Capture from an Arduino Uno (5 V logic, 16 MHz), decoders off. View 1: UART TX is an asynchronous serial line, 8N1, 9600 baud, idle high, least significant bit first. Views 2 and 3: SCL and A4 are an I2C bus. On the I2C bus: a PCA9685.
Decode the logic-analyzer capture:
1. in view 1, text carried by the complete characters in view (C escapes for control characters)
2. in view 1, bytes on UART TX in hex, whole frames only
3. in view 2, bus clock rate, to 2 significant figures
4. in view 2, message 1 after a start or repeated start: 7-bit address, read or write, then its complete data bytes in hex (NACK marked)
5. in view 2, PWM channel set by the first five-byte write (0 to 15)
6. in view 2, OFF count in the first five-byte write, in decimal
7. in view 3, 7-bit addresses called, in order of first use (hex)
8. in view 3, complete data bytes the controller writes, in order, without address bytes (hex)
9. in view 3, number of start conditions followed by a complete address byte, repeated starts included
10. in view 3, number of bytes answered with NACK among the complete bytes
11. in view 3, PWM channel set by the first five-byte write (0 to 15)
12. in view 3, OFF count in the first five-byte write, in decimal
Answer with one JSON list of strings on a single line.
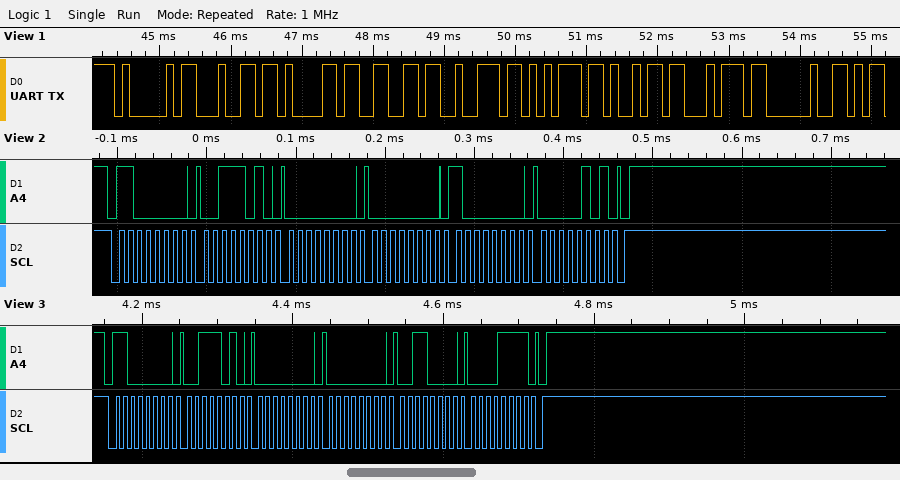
["\"Adafruit \"", "41 64 61 66 72 75 69 74 20", "100 kHz", "0x60 write: 3A 00 00 80 05", "13", "1408", "0x60", "3A 00 00 30 0F", "1", "0", "13", "3888"]
